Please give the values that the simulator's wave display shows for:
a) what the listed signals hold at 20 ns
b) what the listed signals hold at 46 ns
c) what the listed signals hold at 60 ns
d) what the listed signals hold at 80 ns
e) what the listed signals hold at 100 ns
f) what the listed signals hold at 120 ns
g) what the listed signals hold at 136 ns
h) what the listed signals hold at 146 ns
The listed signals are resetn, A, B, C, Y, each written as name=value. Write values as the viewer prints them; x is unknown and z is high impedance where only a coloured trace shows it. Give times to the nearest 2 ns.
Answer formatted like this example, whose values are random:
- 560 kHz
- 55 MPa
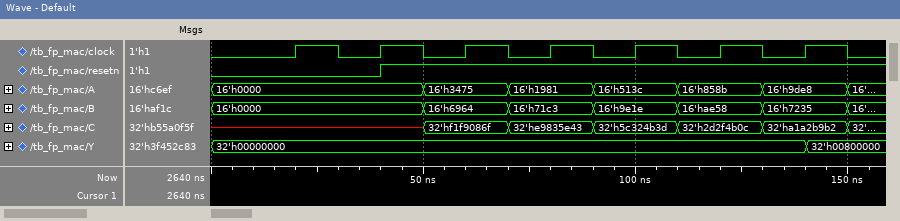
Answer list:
- resetn=0, A=16'h0000, B=16'h0000, C=x, Y=32'h00000000
- resetn=1, A=16'h0000, B=16'h0000, C=x, Y=32'h00000000
- resetn=1, A=16'h3475, B=16'h6964, C=32'hf1f9086f, Y=32'h00000000
- resetn=1, A=16'h1981, B=16'h71c3, C=32'he9835e43, Y=32'h00000000
- resetn=1, A=16'h513c, B=16'h9e1e, C=32'h5c324b3d, Y=32'h00000000
- resetn=1, A=16'h858b, B=16'hae58, C=32'h2d2f4b0c, Y=32'h00000000
- resetn=1, A=16'h9de8, B=16'h7235, C=32'ha1a2b9b2, Y=32'h00000000
- resetn=1, A=16'h9de8, B=16'h7235, C=32'ha1a2b9b2, Y=32'h00800000
